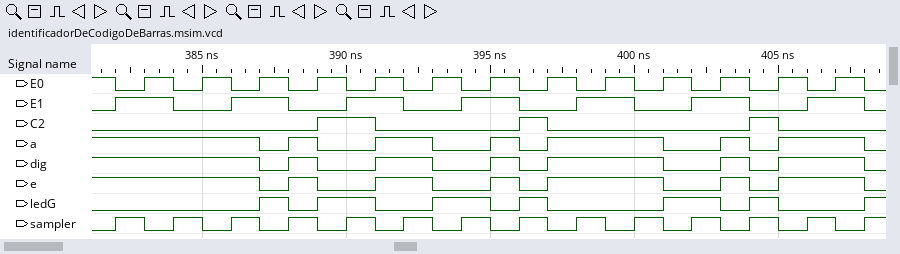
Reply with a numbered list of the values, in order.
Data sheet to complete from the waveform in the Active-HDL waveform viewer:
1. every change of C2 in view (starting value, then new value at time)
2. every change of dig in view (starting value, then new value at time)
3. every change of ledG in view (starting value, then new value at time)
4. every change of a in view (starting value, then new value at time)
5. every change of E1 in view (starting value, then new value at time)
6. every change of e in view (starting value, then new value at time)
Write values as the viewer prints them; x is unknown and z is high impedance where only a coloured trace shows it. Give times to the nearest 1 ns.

1. 0, 1 at 389 ns, 0 at 391 ns, 1 at 396 ns, 0 at 397 ns, 1 at 404 ns, 0 at 405 ns
2. 1, 0 at 387 ns, 1 at 388 ns, 0 at 389 ns, 1 at 391 ns, 0 at 393 ns, 1 at 395 ns, 0 at 396 ns, 1 at 397 ns, 0 at 401 ns, 1 at 403 ns, 0 at 404 ns, 1 at 405 ns, 0 at 408 ns
3. 0, 1 at 387 ns, 0 at 388 ns, 1 at 389 ns, 0 at 391 ns, 1 at 393 ns, 0 at 395 ns, 1 at 396 ns, 0 at 397 ns, 1 at 401 ns, 0 at 403 ns, 1 at 404 ns, 0 at 405 ns, 1 at 408 ns
4. 1, 0 at 387 ns, 1 at 388 ns, 0 at 389 ns, 1 at 391 ns, 0 at 393 ns, 1 at 395 ns, 0 at 396 ns, 1 at 397 ns, 0 at 401 ns, 1 at 403 ns, 0 at 404 ns, 1 at 405 ns, 0 at 408 ns
5. 0, 1 at 382 ns, 0 at 384 ns, 1 at 386 ns, 0 at 388 ns, 1 at 390 ns, 0 at 392 ns, 1 at 394 ns, 0 at 396 ns, 1 at 398 ns, 0 at 400 ns, 1 at 402 ns, 0 at 404 ns, 1 at 406 ns, 0 at 408 ns
6. 1, 0 at 387 ns, 1 at 388 ns, 0 at 389 ns, 1 at 391 ns, 0 at 393 ns, 1 at 395 ns, 0 at 396 ns, 1 at 397 ns, 0 at 401 ns, 1 at 403 ns, 0 at 404 ns, 1 at 405 ns, 0 at 408 ns
